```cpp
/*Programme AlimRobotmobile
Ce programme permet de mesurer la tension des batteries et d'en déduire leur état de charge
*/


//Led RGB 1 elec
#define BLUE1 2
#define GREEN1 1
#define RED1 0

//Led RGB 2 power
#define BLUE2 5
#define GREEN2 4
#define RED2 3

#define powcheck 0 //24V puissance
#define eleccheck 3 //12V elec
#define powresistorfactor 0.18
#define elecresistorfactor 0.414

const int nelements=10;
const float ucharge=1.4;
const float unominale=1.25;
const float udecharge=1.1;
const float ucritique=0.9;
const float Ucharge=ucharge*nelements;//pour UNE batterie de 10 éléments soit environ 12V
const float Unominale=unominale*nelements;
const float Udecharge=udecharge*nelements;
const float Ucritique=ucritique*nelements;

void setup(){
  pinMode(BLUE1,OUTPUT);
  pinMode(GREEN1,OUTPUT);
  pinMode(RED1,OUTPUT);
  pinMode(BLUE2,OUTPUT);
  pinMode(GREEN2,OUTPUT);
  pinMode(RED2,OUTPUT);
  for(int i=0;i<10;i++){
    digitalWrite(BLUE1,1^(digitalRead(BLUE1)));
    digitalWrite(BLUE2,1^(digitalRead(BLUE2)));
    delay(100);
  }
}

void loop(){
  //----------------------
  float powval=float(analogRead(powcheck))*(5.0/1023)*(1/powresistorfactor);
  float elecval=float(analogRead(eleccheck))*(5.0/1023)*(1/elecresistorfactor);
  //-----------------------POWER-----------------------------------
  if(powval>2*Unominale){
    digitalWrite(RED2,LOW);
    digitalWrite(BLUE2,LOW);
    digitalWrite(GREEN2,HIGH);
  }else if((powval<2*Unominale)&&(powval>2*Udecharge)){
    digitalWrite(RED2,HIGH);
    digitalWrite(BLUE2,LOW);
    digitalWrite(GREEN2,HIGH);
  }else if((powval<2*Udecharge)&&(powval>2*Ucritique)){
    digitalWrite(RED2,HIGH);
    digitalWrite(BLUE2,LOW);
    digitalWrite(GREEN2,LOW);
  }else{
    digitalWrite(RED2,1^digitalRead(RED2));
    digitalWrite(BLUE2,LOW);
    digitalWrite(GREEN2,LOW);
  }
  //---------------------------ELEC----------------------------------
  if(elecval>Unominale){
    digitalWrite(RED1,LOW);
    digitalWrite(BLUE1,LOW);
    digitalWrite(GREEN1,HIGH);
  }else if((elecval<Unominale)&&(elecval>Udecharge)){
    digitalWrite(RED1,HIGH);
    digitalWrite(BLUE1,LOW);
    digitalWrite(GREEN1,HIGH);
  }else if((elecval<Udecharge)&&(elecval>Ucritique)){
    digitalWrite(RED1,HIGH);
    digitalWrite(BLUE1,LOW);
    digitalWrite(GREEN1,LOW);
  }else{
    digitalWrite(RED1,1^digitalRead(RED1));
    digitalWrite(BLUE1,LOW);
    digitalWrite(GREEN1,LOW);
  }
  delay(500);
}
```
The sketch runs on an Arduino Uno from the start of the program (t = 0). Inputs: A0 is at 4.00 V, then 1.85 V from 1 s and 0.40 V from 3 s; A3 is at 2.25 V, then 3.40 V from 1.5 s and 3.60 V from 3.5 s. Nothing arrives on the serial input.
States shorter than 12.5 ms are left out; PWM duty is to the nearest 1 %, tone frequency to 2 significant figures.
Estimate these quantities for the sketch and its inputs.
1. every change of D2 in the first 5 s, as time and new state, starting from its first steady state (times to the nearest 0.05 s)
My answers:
0 s high; 0.1 s low; 0.2 s high; 0.3 s low; 0.4 s high; 0.5 s low; 0.6 s high; 0.7 s low; 0.8 s high; 0.9 s low
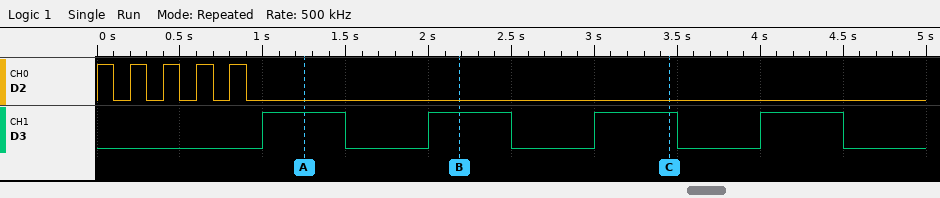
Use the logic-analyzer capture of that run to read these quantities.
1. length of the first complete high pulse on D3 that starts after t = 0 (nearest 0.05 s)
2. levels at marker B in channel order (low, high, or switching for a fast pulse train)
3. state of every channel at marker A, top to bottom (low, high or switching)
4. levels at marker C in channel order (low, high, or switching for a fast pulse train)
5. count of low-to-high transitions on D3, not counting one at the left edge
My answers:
0.50 s
D2 low, D3 high
D2 low, D3 high
D2 low, D3 high
4
